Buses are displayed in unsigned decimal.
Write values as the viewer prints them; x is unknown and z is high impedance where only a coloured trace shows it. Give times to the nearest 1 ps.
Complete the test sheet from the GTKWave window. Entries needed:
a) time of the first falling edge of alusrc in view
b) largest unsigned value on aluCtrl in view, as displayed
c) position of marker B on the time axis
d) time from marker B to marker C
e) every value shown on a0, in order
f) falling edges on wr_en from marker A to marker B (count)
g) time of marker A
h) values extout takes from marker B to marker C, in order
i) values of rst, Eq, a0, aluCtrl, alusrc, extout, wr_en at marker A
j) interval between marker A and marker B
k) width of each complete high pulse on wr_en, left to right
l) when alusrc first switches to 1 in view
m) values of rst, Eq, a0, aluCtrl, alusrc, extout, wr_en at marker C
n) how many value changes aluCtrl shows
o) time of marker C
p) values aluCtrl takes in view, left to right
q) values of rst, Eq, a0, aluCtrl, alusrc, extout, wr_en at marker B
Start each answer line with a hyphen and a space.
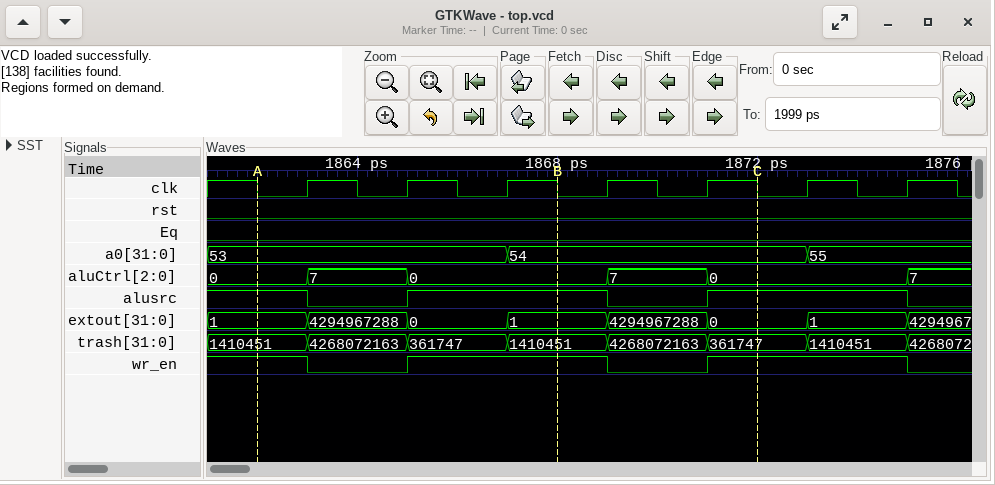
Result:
- 1863 ps
- 7
- 1868 ps
- 4 ps
- 53, 54, 55
- 1
- 1862 ps
- 1, 4294967288, 0
- rst=0, Eq=0, a0=53, aluCtrl=0, alusrc=1, extout=1, wr_en=1
- 6 ps
- 4 ps, 4 ps
- 1865 ps
- rst=0, Eq=0, a0=54, aluCtrl=0, alusrc=1, extout=0, wr_en=1
- 5
- 1872 ps
- 0, 7, 0, 7, 0, 7
- rst=0, Eq=0, a0=54, aluCtrl=0, alusrc=1, extout=1, wr_en=1
